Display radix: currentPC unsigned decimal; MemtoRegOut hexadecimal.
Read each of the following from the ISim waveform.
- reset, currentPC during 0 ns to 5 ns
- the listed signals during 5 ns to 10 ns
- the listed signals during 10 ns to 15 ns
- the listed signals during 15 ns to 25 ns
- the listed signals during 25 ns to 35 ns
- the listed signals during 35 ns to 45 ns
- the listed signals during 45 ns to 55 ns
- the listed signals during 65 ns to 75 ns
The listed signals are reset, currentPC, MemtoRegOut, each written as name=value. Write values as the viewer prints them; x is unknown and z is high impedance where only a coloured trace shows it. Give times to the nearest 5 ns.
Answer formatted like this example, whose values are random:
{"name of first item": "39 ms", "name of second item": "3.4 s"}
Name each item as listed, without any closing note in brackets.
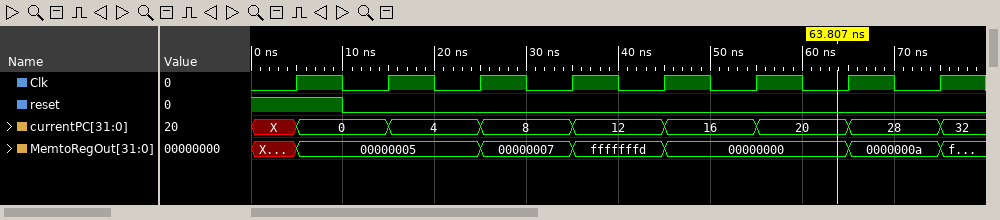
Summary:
{"reset, currentPC during 0 ns to 5 ns": "reset=1, currentPC=X", "the listed signals during 5 ns to 10 ns": "reset=1, currentPC=0, MemtoRegOut=00000005", "the listed signals during 10 ns to 15 ns": "reset=0, currentPC=0, MemtoRegOut=00000005", "the listed signals during 15 ns to 25 ns": "reset=0, currentPC=4, MemtoRegOut=00000005", "the listed signals during 25 ns to 35 ns": "reset=0, currentPC=8, MemtoRegOut=00000007", "the listed signals during 35 ns to 45 ns": "reset=0, currentPC=12, MemtoRegOut=fffffffd", "the listed signals during 45 ns to 55 ns": "reset=0, currentPC=16, MemtoRegOut=00000000", "the listed signals during 65 ns to 75 ns": "reset=0, currentPC=28, MemtoRegOut=0000000a"}
